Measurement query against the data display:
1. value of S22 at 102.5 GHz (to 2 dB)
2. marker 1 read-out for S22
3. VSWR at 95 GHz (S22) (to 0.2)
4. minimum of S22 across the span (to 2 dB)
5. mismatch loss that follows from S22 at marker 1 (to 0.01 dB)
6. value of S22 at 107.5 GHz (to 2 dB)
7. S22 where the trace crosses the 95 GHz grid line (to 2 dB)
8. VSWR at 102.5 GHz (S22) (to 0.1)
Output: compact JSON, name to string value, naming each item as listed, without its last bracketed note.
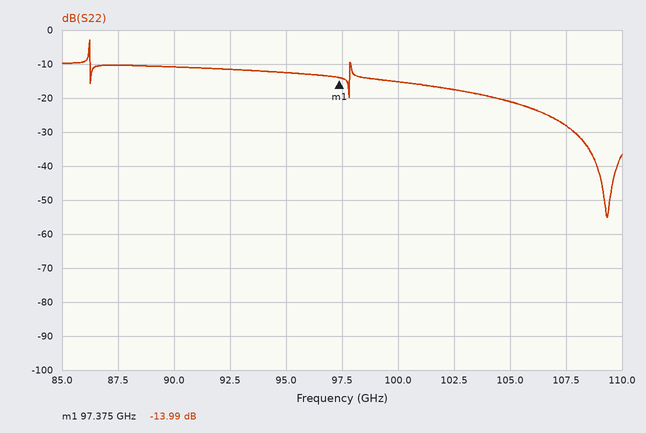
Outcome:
{"value of S22 at 102.5 GHz": "-18 dB", "marker 1 read-out for S22": "-13.99 dB", "VSWR at 95 GHz (S22)": "1.6", "minimum of S22 across the span": "-56 dB", "mismatch loss that follows from S22 at marker 1": "0.18 dB", "value of S22 at 107.5 GHz": "-28 dB", "S22 where the trace crosses the 95 GHz grid line": "-12 dB", "VSWR at 102.5 GHz (S22)": "1.3"}
